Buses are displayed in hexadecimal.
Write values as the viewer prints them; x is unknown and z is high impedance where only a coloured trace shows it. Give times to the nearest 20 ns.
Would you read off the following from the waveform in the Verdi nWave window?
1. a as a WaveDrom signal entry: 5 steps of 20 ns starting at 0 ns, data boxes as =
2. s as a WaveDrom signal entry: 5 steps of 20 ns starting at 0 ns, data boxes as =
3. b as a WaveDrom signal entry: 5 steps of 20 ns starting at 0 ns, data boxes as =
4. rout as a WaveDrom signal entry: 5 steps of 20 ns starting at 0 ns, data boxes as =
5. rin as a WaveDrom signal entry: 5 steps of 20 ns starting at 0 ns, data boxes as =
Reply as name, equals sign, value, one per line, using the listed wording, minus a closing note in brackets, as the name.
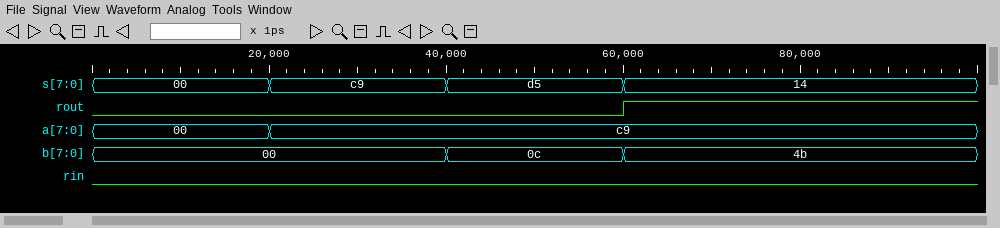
a as a WaveDrom signal entry: 5 steps of 20 ns starting at 0 ns, data boxes as = = {name: 'a', wave: '==...', data: '00 c9'}
s as a WaveDrom signal entry: 5 steps of 20 ns starting at 0 ns, data boxes as = = {name: 's', wave: '====.', data: '00 c9 d5 14'}
b as a WaveDrom signal entry: 5 steps of 20 ns starting at 0 ns, data boxes as = = {name: 'b', wave: '=.==.', data: '00 0c 4b'}
rout as a WaveDrom signal entry: 5 steps of 20 ns starting at 0 ns, data boxes as = = {name: 'rout', wave: '0..1.'}
rin as a WaveDrom signal entry: 5 steps of 20 ns starting at 0 ns, data boxes as = = {name: 'rin', wave: '0....'}
